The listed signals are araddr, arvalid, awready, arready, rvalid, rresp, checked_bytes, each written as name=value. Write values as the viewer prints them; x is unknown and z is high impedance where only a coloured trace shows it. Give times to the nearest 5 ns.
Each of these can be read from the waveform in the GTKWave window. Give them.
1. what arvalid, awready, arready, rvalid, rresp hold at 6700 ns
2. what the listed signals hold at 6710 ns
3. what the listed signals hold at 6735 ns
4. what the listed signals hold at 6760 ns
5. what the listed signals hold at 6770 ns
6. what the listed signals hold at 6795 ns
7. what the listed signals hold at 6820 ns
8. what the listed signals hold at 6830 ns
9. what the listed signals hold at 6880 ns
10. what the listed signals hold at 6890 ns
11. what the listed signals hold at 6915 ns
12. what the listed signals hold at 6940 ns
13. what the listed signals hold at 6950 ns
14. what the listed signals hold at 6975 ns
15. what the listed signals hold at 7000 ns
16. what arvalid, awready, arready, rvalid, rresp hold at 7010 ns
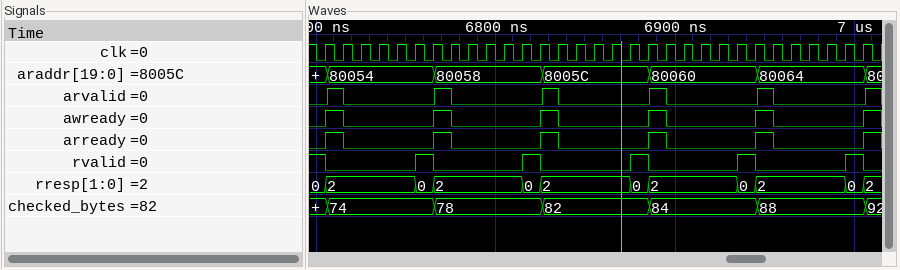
arvalid=0, awready=0, arready=0, rvalid=1, rresp=0
araddr=80054, arvalid=1, awready=1, arready=1, rvalid=0, rresp=2, checked_bytes=74
araddr=80054, arvalid=0, awready=0, arready=0, rvalid=0, rresp=2, checked_bytes=74
araddr=80054, arvalid=0, awready=0, arready=0, rvalid=1, rresp=0, checked_bytes=74
araddr=80058, arvalid=1, awready=1, arready=1, rvalid=0, rresp=2, checked_bytes=78
araddr=80058, arvalid=0, awready=0, arready=0, rvalid=0, rresp=2, checked_bytes=78
araddr=80058, arvalid=0, awready=0, arready=0, rvalid=1, rresp=0, checked_bytes=78
araddr=8005C, arvalid=1, awready=1, arready=1, rvalid=0, rresp=2, checked_bytes=82
araddr=8005C, arvalid=0, awready=0, arready=0, rvalid=1, rresp=0, checked_bytes=82
araddr=80060, arvalid=1, awready=1, arready=1, rvalid=0, rresp=2, checked_bytes=84
araddr=80060, arvalid=0, awready=0, arready=0, rvalid=0, rresp=2, checked_bytes=84
araddr=80060, arvalid=0, awready=0, arready=0, rvalid=1, rresp=0, checked_bytes=84
araddr=80064, arvalid=1, awready=1, arready=1, rvalid=0, rresp=2, checked_bytes=88
araddr=80064, arvalid=0, awready=0, arready=0, rvalid=0, rresp=2, checked_bytes=88
araddr=80064, arvalid=0, awready=0, arready=0, rvalid=1, rresp=0, checked_bytes=88
arvalid=1, awready=1, arready=1, rvalid=0, rresp=2
